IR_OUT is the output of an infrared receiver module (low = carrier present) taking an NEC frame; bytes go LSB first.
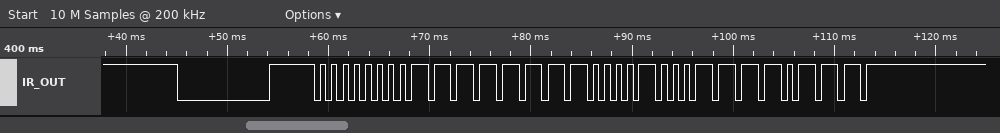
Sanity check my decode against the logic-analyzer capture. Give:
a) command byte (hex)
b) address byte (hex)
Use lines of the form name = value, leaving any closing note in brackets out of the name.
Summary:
command byte = 0x10
address byte = 0x00
